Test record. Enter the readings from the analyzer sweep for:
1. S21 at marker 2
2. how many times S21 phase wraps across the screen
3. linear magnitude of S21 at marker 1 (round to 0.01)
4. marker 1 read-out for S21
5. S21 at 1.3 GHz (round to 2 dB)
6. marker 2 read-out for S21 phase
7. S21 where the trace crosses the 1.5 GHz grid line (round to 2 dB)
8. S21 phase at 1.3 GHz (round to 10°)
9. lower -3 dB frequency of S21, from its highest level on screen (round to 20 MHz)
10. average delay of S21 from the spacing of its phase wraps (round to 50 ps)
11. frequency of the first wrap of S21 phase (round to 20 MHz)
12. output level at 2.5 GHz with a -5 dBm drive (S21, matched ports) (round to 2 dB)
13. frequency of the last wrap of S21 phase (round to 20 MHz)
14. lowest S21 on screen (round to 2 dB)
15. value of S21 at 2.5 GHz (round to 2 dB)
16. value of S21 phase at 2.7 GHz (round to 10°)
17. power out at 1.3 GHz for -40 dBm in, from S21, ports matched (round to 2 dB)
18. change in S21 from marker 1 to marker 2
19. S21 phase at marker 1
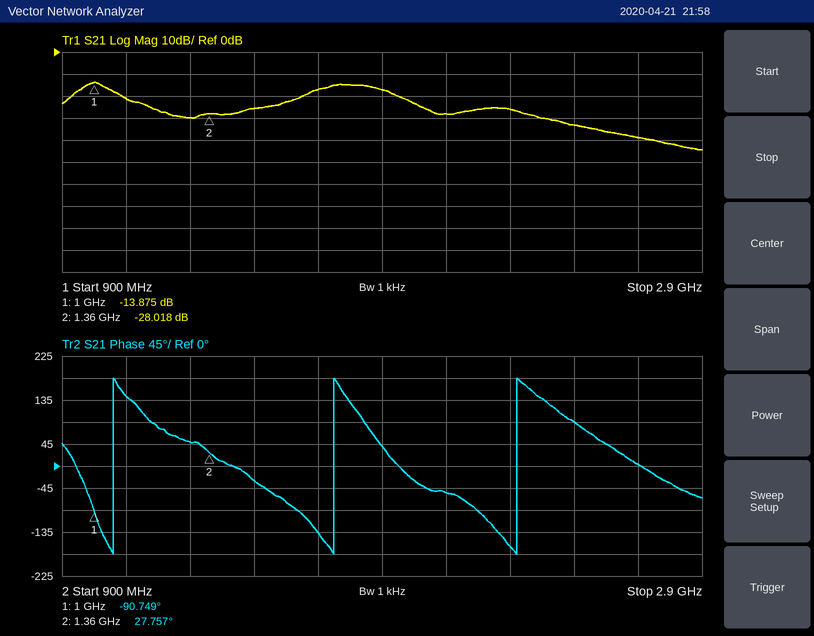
-28.018 dB
3
0.20
-13.875 dB
-30 dB
27.757°
-26 dB
50°
960 MHz
1.60 ns
1.06 GHz
-38 dBm
2.32 GHz
-44 dB
-34 dB
0°
-70 dBm
-14.143 dB
-90.749°
